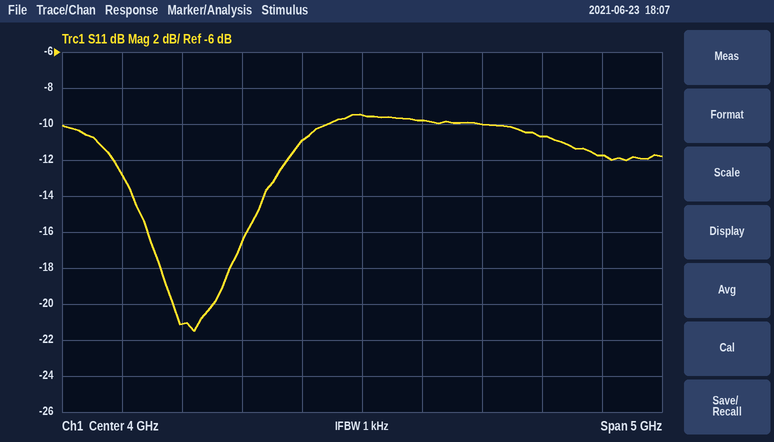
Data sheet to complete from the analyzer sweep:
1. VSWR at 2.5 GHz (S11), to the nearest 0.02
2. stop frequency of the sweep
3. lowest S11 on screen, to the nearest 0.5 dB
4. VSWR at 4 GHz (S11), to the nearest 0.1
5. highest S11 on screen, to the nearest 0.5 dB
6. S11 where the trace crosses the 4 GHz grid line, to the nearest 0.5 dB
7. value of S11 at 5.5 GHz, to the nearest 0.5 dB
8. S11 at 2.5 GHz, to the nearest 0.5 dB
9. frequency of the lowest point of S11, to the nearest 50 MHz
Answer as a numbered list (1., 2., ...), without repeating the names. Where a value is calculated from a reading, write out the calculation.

1. |Γ| = 10^(-21/20) = 0.0891; VSWR = (1 + 0.0891)/(1 − 0.0891) ≈ 1.20
2. 6.5 GHz
3. -21.5 dB
4. |Γ| = 10^(-9.5/20) = 0.3350; VSWR = (1 + 0.3350)/(1 − 0.3350) ≈ 2.0
5. -9.5 dB
6. -9.5 dB
7. -10.5 dB
8. -21.0 dB
9. 2.60 GHz
